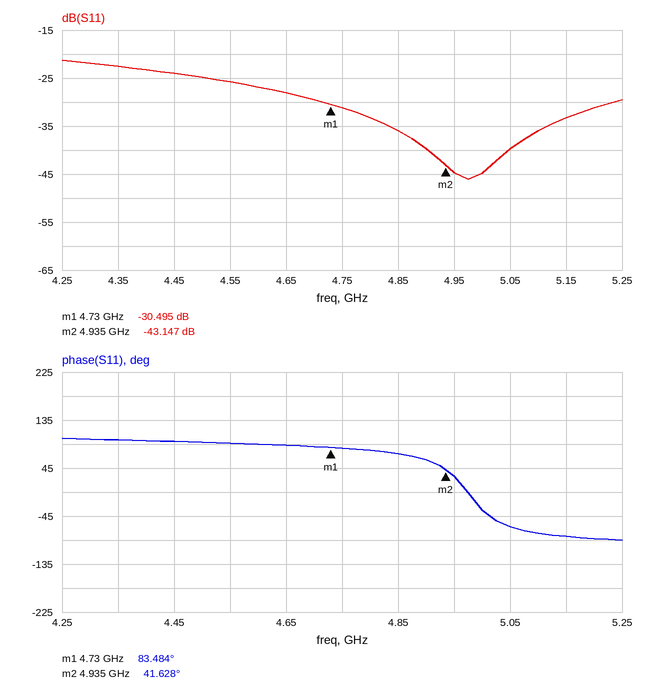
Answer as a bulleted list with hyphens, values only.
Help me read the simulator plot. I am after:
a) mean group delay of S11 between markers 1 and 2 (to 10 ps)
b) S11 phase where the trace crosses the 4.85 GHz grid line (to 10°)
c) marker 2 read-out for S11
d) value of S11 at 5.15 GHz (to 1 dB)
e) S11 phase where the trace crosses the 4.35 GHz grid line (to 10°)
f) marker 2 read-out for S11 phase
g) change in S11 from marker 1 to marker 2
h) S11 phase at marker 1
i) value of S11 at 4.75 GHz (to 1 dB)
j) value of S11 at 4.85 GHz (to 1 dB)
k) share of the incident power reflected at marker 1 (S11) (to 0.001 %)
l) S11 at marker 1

- 570 ps
- 70°
- -43.147 dB
- -33 dB
- 100°
- 41.628°
- -12.652 dB
- 83.484°
- -31 dB
- -36 dB
- 0.089 %
- -30.495 dB
